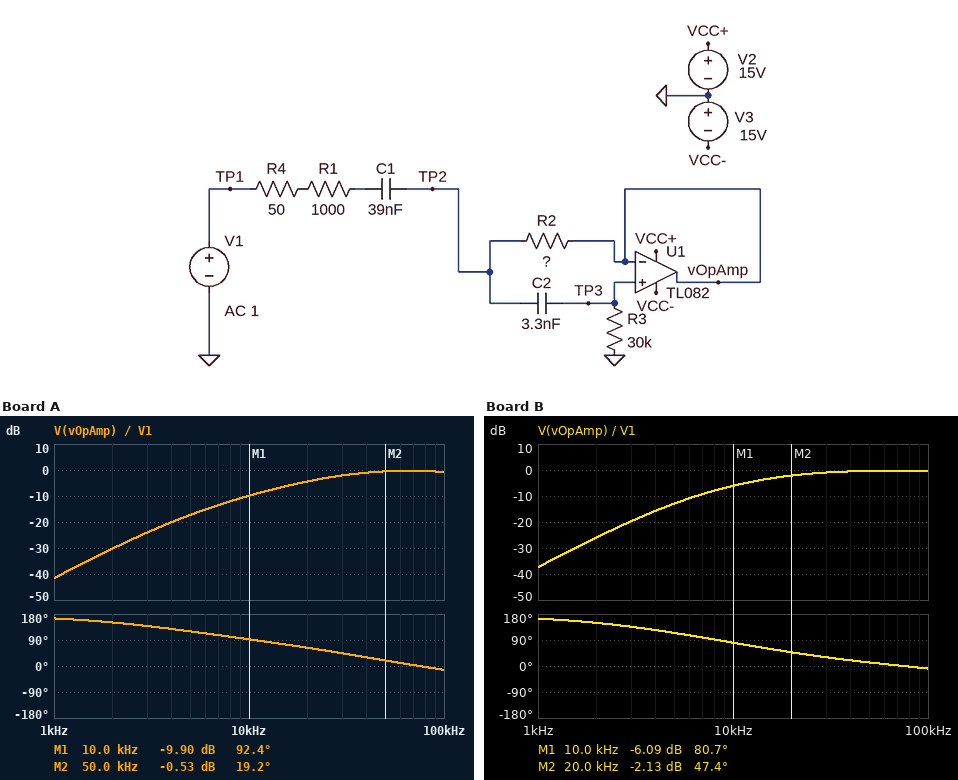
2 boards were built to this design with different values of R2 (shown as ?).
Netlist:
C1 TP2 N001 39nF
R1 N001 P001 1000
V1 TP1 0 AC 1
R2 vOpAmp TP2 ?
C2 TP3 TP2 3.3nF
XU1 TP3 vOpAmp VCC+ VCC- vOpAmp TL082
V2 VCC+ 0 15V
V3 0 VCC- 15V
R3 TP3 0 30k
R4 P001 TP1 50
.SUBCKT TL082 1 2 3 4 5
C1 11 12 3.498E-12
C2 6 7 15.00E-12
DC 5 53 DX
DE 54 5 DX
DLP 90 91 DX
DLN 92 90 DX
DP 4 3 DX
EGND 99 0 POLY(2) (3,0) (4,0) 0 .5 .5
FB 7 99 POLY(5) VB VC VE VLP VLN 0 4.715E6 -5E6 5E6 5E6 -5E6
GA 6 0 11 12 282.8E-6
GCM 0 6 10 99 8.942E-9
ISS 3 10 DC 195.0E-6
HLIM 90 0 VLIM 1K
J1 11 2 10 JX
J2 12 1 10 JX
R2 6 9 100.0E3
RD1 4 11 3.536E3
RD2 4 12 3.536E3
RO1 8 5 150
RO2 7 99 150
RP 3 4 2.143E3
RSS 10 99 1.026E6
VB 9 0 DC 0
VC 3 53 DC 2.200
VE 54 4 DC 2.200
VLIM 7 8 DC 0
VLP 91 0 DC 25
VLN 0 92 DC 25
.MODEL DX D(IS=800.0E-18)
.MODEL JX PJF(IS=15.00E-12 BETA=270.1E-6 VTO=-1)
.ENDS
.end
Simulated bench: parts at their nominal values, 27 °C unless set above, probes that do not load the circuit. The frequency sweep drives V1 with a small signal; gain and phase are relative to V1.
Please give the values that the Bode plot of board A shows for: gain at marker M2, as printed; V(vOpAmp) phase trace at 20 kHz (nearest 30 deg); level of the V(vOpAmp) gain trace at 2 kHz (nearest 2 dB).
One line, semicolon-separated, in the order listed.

-0.53 dB; 60 deg; -30 dB
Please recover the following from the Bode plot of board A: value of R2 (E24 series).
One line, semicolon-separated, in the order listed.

56 Ω
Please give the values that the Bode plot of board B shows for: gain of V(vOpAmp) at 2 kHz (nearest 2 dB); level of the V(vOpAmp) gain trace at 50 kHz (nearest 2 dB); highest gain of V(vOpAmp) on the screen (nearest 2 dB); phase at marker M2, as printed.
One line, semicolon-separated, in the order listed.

-26 dB; 0 dB; 0 dB; 47.4 deg
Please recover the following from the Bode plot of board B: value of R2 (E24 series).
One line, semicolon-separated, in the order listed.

91 Ω
